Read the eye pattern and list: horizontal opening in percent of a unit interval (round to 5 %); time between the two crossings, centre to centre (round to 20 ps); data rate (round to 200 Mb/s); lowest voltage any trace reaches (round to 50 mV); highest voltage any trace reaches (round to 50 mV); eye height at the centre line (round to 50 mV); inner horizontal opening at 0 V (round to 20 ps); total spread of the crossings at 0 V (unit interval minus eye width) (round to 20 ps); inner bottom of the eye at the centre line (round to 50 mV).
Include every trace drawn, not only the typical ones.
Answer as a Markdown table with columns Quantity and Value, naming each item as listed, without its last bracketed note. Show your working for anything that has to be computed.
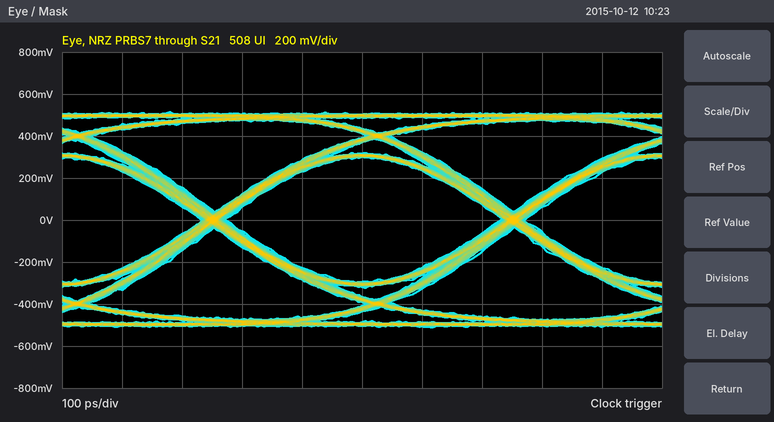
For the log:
| Quantity | Value |
|---|---|
| horizontal opening in percent of a unit interval | 460 ps / 500 ps ≈ 92.0 %, so 90 % to the nearest 5 % |
| time between the two crossings, centre to centre | 500 ps |
| data rate | 2.0 Gb/s |
| lowest voltage any trace reaches | -500 mV |
| highest voltage any trace reaches | 500 mV |
| eye height at the centre line | 600 mV |
| inner horizontal opening at 0 V | 460 ps |
| total spread of the crossings at 0 V (unit interval minus eye width) | 40 ps |
| inner bottom of the eye at the centre line | -300 mV |
